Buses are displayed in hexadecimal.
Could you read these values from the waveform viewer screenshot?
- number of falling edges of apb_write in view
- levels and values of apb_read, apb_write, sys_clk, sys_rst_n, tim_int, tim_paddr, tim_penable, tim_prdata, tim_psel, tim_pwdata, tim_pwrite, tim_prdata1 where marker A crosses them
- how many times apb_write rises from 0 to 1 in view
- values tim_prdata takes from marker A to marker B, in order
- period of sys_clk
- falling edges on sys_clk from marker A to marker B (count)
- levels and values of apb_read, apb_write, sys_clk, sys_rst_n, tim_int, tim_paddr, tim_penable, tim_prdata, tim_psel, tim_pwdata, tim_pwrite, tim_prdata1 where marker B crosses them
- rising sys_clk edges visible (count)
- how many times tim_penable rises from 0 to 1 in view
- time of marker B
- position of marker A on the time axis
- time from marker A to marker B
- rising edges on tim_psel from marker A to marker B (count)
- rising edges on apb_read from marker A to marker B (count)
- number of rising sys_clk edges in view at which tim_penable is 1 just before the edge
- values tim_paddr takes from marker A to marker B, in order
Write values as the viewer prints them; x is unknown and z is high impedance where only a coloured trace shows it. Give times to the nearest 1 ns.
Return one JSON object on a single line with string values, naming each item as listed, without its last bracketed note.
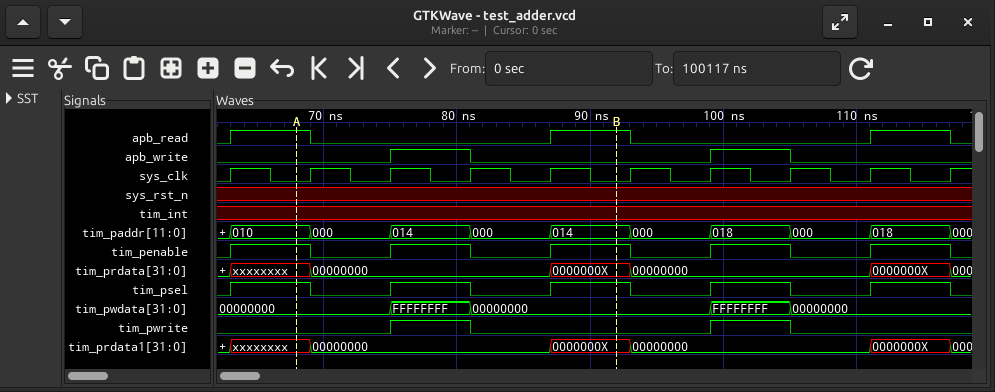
{"number of falling edges of apb_write in view": "2", "levels and values of apb_read, apb_write, sys_clk, sys_rst_n, tim_int, tim_paddr, tim_penable, tim_prdata, tim_psel, tim_pwdata, tim_pwrite, tim_prdata1 where marker A crosses them": "apb_read=1, apb_write=0, sys_clk=0, sys_rst_n=x, tim_int=x, tim_paddr=010, tim_penable=1, tim_prdata=xxxxxxxx, tim_psel=1, tim_pwdata=00000000, tim_pwrite=0, tim_prdata1=xxxxxxxx", "how many times apb_write rises from 0 to 1 in view": "2", "values tim_prdata takes from marker A to marker B, in order": "xxxxxxxx, 00000000, 0000000X", "period of sys_clk": "6 ns", "falling edges on sys_clk from marker A to marker B": "4", "levels and values of apb_read, apb_write, sys_clk, sys_rst_n, tim_int, tim_paddr, tim_penable, tim_prdata, tim_psel, tim_pwdata, tim_pwrite, tim_prdata1 where marker B crosses them": "apb_read=1, apb_write=0, sys_clk=0, sys_rst_n=x, tim_int=x, tim_paddr=014, tim_penable=1, tim_prdata=0000000X, tim_psel=1, tim_pwdata=00000000, tim_pwrite=0, tim_prdata1=0000000X", "rising sys_clk edges visible": "10", "how many times tim_penable rises from 0 to 1 in view": "5", "time of marker B": "92 ns", "position of marker A on the time axis": "68 ns", "time from marker A to marker B": "24 ns", "rising edges on tim_psel from marker A to marker B": "2", "rising edges on apb_read from marker A to marker B": "1", "number of rising sys_clk edges in view at which tim_penable is 1 just before the edge": "5", "values tim_paddr takes from marker A to marker B, in order": "010, 000, 014, 000, 014"}
